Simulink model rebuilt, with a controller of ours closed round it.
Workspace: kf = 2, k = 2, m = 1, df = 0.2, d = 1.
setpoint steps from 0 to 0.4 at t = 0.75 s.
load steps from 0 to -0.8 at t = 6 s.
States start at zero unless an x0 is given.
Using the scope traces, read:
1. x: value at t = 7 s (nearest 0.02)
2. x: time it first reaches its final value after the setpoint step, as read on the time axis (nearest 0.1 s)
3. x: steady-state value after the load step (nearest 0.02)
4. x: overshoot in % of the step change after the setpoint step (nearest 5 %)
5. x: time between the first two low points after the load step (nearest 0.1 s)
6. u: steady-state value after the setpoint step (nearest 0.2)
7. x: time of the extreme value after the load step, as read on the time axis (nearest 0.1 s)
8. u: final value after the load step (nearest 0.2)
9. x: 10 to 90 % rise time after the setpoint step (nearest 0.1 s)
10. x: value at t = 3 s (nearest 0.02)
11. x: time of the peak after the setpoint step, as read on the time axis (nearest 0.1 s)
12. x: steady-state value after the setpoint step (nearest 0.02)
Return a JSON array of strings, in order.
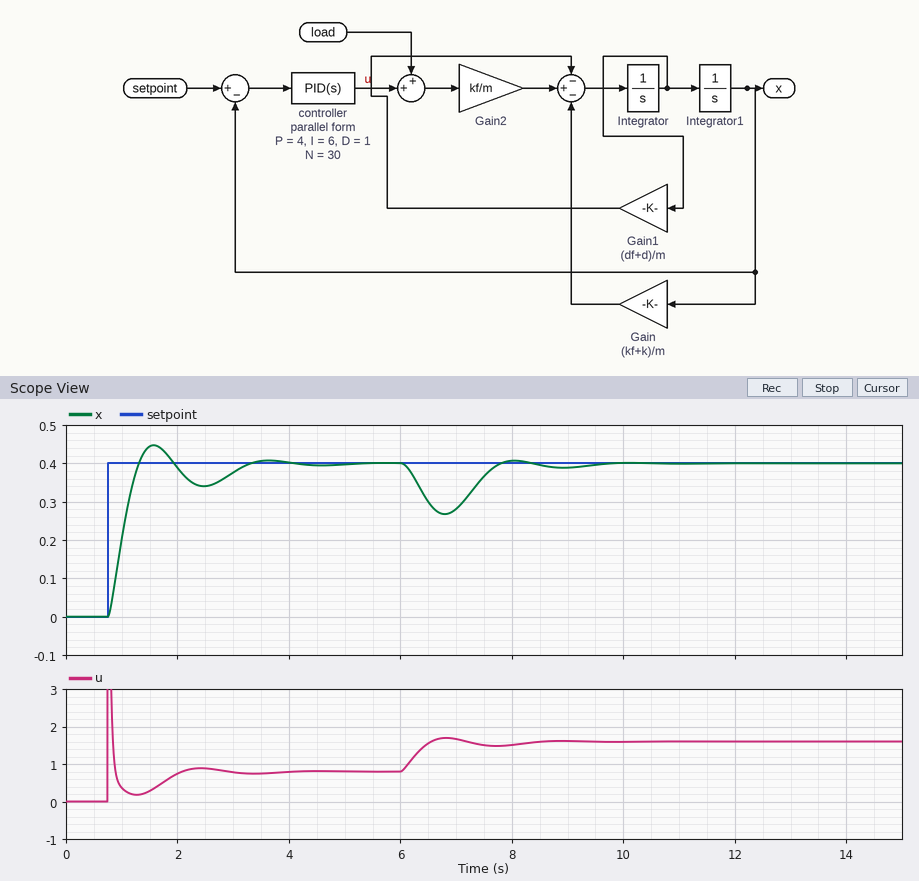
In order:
["0.28", "1.3 s", "0.40", "10 %", "2.1 s", "0.8", "6.8 s", "1.6", "0.4 s", "0.38", "1.6 s", "0.40"]
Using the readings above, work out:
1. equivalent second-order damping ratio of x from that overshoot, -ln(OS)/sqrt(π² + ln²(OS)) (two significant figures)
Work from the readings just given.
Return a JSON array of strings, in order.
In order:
["0.59"]
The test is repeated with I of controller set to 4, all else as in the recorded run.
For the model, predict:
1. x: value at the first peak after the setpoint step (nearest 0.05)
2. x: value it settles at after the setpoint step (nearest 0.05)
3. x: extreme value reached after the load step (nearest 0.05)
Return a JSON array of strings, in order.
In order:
["0.40", "0.40", "0.25"]
